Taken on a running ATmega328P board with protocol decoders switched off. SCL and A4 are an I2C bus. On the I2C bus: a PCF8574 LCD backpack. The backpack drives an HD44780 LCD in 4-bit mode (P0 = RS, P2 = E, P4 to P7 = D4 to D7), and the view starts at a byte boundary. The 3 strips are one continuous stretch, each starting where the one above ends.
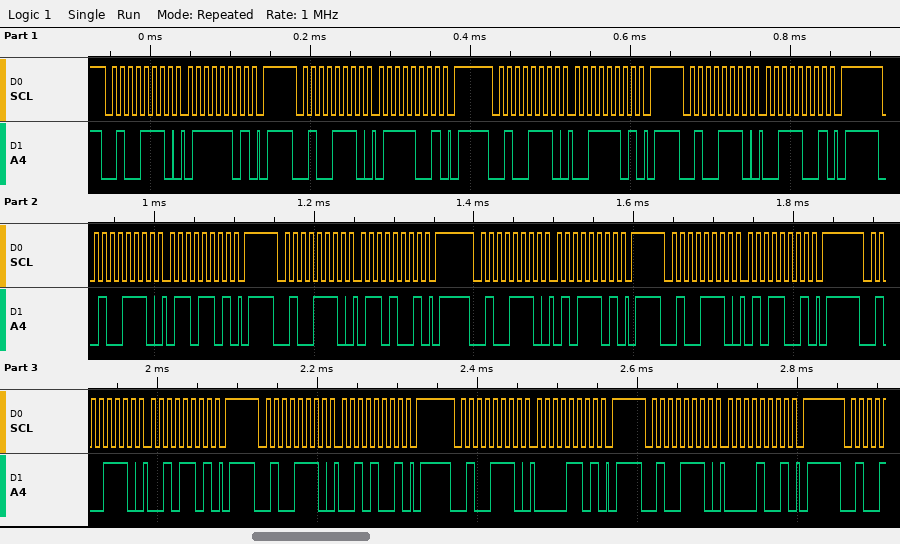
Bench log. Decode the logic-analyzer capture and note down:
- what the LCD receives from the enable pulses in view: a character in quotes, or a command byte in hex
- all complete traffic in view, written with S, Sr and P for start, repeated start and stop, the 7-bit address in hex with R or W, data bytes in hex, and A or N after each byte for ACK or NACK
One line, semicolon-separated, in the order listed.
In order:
's' 'e' ' '; S 27W A 7D A P S 27W A 79 A P S 27W A 3D A P S 27W A 39 A P S 27W A 6D A P S 27W A 69 A P S 27W A 5D A P S 27W A 59 A P S 27W A 2D A P S 27W A 29 A P S 27W A 0D A P S 27W A 09 A P
